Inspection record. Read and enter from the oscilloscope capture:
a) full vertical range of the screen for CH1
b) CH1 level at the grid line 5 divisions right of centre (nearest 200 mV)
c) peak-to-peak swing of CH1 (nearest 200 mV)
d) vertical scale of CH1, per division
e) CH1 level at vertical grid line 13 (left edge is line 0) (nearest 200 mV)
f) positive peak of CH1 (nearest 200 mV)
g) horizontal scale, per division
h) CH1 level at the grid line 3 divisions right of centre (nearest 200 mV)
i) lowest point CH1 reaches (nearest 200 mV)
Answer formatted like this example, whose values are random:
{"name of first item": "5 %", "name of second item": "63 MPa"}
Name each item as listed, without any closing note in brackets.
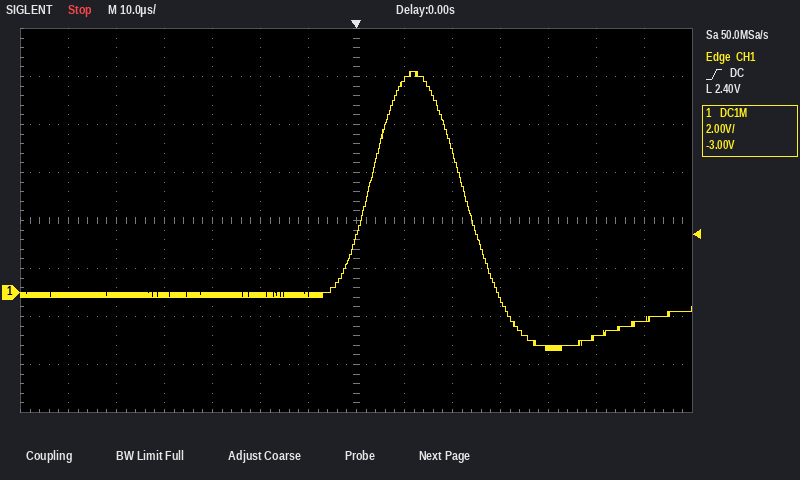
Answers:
{"full vertical range of the screen for CH1": "16 V", "CH1 level at the grid line 5 divisions right of centre": "-1.8 V", "peak-to-peak swing of CH1": "11.6 V", "vertical scale of CH1, per division": "2 V", "CH1 level at vertical grid line 13 (left edge is line 0)": "-1.2 V", "positive peak of CH1": "9.2 V", "horizontal scale, per division": "10 µs", "CH1 level at the grid line 3 divisions right of centre": "-200 mV", "lowest point CH1 reaches": "-2.4 V"}
